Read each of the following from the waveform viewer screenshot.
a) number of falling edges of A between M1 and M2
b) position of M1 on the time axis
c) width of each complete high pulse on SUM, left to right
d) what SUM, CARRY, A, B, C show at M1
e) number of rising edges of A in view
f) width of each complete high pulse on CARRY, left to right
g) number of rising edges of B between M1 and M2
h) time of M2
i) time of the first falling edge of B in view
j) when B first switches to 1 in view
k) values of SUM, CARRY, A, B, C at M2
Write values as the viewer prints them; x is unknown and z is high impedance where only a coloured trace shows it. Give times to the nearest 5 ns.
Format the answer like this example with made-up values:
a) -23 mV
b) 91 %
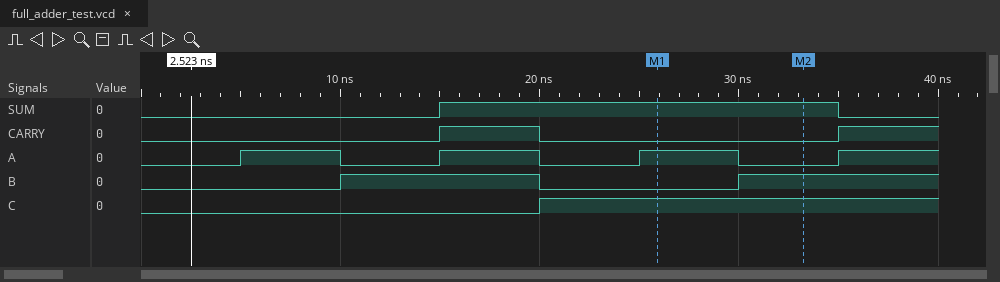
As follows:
a) 1
b) 25 ns
c) 20 ns
d) SUM=1, CARRY=0, A=1, B=0, C=1
e) 4
f) 5 ns
g) 1
h) 35 ns
i) 20 ns
j) 10 ns
k) SUM=1, CARRY=0, A=0, B=1, C=1
